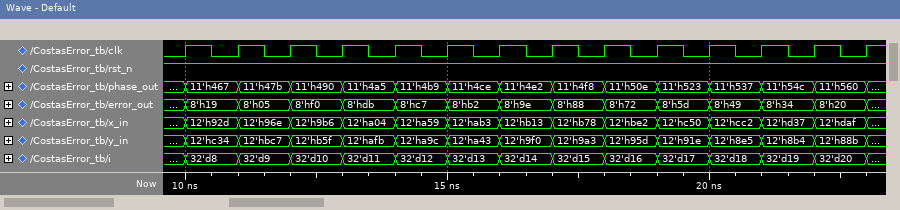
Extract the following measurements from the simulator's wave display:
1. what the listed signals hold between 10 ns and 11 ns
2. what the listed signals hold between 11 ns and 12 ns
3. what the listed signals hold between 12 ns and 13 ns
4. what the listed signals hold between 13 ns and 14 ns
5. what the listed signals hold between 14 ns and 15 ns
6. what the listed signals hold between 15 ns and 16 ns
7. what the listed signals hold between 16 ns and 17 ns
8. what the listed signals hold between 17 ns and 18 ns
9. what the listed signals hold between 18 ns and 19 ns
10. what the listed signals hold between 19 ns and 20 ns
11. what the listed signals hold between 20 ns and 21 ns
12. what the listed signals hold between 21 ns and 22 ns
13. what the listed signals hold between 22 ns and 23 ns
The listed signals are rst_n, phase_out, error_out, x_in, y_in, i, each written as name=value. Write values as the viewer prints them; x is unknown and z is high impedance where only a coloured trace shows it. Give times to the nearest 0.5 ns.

rst_n=1, phase_out=11'h467, error_out=8'h19, x_in=12'h92d, y_in=12'hc34, i=32'd8
rst_n=1, phase_out=11'h47b, error_out=8'h05, x_in=12'h96e, y_in=12'hbc7, i=32'd9
rst_n=1, phase_out=11'h490, error_out=8'hf0, x_in=12'h9b6, y_in=12'hb5f, i=32'd10
rst_n=1, phase_out=11'h4a5, error_out=8'hdb, x_in=12'ha04, y_in=12'hafb, i=32'd11
rst_n=1, phase_out=11'h4b9, error_out=8'hc7, x_in=12'ha59, y_in=12'ha9c, i=32'd12
rst_n=1, phase_out=11'h4ce, error_out=8'hb2, x_in=12'hab3, y_in=12'ha43, i=32'd13
rst_n=1, phase_out=11'h4e2, error_out=8'h9e, x_in=12'hb13, y_in=12'h9f0, i=32'd14
rst_n=1, phase_out=11'h4f8, error_out=8'h88, x_in=12'hb78, y_in=12'h9a3, i=32'd15
rst_n=1, phase_out=11'h50e, error_out=8'h72, x_in=12'hbe2, y_in=12'h95d, i=32'd16
rst_n=1, phase_out=11'h523, error_out=8'h5d, x_in=12'hc50, y_in=12'h91e, i=32'd17
rst_n=1, phase_out=11'h537, error_out=8'h49, x_in=12'hcc2, y_in=12'h8e5, i=32'd18
rst_n=1, phase_out=11'h54c, error_out=8'h34, x_in=12'hd37, y_in=12'h8b4, i=32'd19
rst_n=1, phase_out=11'h560, error_out=8'h20, x_in=12'hdaf, y_in=12'h88b, i=32'd20
